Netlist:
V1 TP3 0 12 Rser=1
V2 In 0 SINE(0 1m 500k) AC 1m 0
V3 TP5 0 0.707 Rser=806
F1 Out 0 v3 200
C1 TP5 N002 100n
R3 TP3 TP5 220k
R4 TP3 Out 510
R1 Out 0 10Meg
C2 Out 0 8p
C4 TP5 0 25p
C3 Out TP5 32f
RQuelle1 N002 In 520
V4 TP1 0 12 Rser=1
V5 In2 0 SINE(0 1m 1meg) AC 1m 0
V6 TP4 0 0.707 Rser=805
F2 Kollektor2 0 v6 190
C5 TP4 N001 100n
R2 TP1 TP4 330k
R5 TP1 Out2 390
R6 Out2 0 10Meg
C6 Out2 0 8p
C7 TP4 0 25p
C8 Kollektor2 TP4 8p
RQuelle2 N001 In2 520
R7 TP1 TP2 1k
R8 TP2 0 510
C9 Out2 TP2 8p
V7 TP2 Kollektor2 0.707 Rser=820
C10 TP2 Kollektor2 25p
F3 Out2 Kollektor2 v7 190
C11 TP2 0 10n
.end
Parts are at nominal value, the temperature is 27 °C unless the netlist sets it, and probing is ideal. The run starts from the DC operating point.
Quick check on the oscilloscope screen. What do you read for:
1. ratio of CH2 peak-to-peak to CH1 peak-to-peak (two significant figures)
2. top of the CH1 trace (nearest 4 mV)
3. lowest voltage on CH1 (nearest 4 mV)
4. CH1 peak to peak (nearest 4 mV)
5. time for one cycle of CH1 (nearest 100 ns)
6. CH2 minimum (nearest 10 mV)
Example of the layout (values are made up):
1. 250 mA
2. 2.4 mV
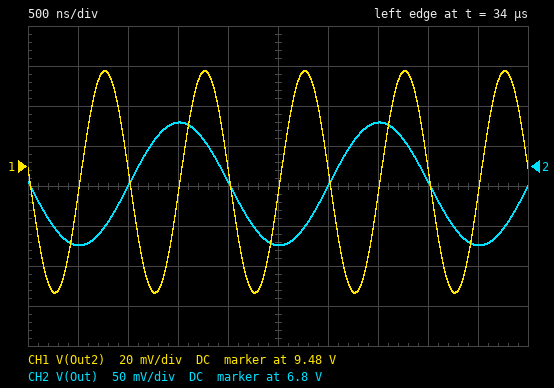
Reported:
1. 1.4
2. 9.528 V
3. 9.416 V
4. 112 mV
5. 1.0 µs
6. 6.70 V
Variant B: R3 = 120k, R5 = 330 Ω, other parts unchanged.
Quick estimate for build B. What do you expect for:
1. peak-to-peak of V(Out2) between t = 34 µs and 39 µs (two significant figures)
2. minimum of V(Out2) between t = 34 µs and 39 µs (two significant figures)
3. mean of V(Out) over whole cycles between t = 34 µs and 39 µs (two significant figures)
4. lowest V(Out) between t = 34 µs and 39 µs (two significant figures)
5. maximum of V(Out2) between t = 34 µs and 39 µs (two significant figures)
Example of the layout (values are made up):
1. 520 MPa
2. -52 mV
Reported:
1. 94 mV
2. 9.8 V
3. 2.5 V
4. 2.4 V
5. 9.9 V
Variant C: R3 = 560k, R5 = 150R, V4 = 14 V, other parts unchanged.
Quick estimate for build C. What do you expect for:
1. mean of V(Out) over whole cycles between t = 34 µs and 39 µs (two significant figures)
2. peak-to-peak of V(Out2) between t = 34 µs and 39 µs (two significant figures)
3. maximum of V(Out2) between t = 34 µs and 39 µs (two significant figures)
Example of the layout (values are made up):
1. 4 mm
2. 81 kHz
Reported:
1. 9.9 V
2. 43 mV
3. 13 V
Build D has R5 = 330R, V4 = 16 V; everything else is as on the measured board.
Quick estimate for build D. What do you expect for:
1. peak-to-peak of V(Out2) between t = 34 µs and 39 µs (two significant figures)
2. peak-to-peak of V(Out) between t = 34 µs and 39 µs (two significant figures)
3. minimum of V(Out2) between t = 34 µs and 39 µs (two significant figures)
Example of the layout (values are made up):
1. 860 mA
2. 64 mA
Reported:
1. 94 mV
2. 150 mV
3. 13 V
